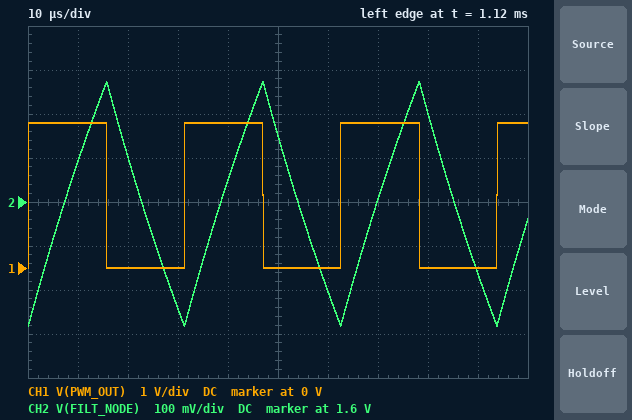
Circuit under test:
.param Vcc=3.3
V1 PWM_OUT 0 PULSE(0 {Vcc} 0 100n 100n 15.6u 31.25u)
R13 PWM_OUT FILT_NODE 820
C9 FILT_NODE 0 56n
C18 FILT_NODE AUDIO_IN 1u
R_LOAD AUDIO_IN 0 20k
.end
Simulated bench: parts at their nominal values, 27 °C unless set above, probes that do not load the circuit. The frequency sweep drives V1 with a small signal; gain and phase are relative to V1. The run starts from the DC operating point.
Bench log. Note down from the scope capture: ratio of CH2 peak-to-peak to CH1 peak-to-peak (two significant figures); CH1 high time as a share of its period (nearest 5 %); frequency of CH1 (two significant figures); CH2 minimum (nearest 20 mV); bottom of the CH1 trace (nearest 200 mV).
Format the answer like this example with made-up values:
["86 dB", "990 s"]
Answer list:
["0.17", "50 %", "32 kHz", "1.32 V", "0 V"]
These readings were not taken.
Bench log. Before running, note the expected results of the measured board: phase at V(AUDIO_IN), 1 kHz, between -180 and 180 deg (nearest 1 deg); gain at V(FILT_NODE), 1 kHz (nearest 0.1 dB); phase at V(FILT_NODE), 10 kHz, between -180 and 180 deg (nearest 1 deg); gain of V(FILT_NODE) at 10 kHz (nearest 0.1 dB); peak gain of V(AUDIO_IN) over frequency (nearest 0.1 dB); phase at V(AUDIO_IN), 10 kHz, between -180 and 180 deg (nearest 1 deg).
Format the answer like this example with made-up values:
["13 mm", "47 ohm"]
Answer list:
["-15 deg", "-0.7 dB", "-70 deg", "-9.7 dB", "-0.4 dB", "-70 deg"]
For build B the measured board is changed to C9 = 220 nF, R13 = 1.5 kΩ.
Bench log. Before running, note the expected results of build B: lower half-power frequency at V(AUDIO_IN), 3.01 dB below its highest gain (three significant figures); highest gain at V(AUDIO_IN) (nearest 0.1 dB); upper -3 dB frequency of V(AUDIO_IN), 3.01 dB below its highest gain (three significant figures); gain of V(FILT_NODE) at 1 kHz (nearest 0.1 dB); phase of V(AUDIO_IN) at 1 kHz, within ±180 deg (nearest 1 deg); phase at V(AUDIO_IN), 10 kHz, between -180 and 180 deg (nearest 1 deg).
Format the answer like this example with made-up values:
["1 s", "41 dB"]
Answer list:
["7.19 Hz", "-0.8 dB", "534 Hz", "-7.4 dB", "-62 deg", "-87 deg"]
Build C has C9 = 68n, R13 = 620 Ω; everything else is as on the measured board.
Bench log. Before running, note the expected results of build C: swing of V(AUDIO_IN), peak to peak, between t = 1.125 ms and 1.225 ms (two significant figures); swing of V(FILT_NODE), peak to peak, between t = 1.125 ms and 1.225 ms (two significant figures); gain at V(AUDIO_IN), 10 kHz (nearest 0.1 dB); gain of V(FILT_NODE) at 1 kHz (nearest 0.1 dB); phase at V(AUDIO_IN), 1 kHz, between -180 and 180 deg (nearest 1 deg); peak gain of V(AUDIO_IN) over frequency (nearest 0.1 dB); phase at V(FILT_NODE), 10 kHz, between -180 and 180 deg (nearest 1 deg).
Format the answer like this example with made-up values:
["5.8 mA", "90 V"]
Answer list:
["610 mV", "600 mV", "-9.1 dB", "-0.5 dB", "-14 deg", "-0.3 dB", "-69 deg"]
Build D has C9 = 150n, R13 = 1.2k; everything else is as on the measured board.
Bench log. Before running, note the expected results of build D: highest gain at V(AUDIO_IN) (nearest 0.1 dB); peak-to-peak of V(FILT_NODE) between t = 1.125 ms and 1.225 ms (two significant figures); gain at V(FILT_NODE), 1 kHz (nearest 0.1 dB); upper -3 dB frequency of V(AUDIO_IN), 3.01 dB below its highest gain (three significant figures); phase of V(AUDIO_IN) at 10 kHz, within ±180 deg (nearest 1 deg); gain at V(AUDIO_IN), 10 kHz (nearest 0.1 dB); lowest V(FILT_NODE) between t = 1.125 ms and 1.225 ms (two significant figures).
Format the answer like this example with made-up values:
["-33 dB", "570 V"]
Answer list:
["-0.6 dB", "140 mV", "-3.8 dB", "953 Hz", "-85 deg", "-21.1 dB", "1.5 V"]
